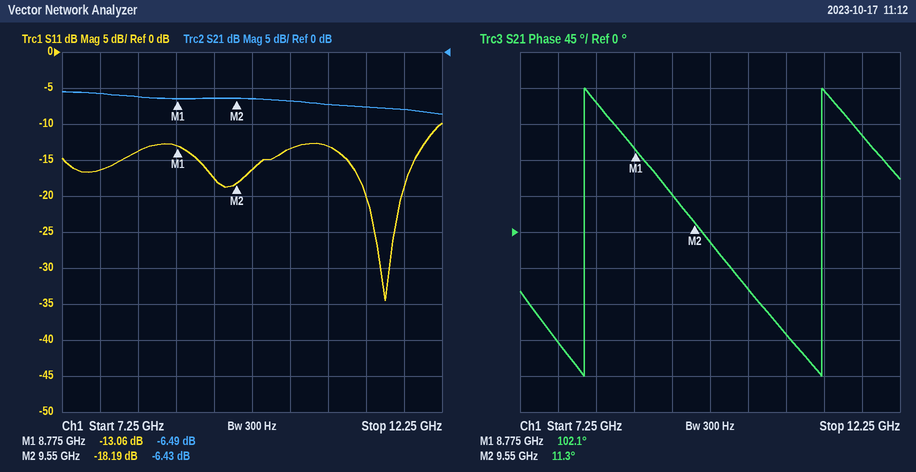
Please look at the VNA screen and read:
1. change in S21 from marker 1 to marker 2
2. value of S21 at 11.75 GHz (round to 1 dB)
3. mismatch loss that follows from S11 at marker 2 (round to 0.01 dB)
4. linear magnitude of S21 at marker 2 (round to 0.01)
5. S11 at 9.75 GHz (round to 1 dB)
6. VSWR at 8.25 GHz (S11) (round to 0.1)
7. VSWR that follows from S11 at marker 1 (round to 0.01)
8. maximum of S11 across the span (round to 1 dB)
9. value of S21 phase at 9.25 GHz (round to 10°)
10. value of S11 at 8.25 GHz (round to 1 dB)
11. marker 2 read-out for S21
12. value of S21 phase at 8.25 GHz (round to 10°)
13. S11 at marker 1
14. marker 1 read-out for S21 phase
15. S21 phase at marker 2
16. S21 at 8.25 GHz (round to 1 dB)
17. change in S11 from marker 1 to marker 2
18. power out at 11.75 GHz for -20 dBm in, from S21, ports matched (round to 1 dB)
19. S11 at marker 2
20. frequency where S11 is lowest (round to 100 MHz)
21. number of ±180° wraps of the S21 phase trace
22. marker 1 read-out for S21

0.06 dB
-8 dB
0.07 dB
0.48
-16 dB
1.5
1.57
-10 dB
50°
-14 dB
-6.43 dB
160°
-13.06 dB
102.1°
11.3°
-6 dB
-5.13 dB
-28 dBm
-18.19 dB
11.5 GHz
2
-6.49 dB
